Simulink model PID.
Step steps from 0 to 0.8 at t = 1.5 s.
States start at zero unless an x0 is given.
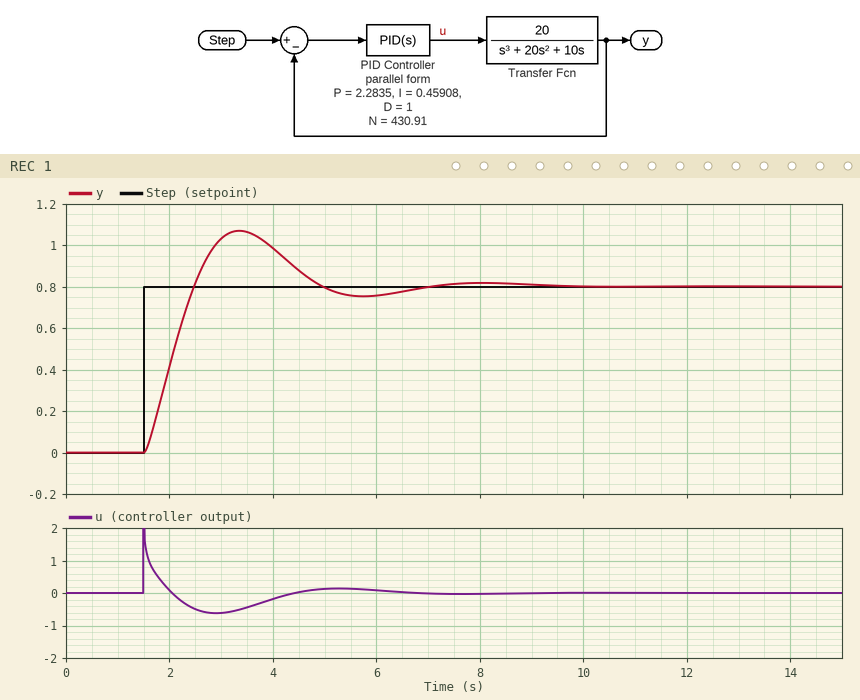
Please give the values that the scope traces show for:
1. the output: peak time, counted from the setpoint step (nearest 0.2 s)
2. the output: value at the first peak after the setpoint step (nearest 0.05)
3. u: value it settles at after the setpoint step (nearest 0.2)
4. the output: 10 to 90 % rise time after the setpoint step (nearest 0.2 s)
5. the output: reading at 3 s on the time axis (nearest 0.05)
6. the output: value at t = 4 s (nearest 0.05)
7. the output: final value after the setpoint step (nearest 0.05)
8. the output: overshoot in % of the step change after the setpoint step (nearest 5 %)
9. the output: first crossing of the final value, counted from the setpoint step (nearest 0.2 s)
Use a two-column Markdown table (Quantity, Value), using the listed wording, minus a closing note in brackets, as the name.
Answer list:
| Quantity | Value |
|---|---|
| the output: peak time, counted from the setpoint step | 1.8 s |
| the output: value at the first peak after the setpoint step | 1.05 |
| u: value it settles at after the setpoint step | 0.0 |
| the output: 10 to 90 % rise time after the setpoint step | 0.8 s |
| the output: reading at 3 s on the time axis | 1.05 |
| the output: value at t = 4 s | 1.00 |
| the output: final value after the setpoint step | 0.80 |
| the output: overshoot in % of the step change after the setpoint step | 35 % |
| the output: first crossing of the final value, counted from the setpoint step | 1.0 s |
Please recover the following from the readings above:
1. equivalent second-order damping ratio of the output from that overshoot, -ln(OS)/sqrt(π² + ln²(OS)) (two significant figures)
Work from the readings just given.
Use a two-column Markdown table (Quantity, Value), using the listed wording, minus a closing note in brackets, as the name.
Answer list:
| Quantity | Value |
|---|---|
| equivalent second-order damping ratio of the output from that overshoot, -ln(OS)/sqrt(π² + ln²(OS)) | 0.32 |
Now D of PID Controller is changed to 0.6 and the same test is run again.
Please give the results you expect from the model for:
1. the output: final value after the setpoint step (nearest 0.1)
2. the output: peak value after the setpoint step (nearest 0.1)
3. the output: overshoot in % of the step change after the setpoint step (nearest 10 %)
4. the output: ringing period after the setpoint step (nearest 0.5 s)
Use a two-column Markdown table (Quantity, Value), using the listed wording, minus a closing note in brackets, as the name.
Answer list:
| Quantity | Value |
|---|---|
| the output: final value after the setpoint step | 0.8 |
| the output: peak value after the setpoint step | 1.2 |
| the output: overshoot in % of the step change after the setpoint step | 50 % |
| the output: ringing period after the setpoint step | 4.5 s |
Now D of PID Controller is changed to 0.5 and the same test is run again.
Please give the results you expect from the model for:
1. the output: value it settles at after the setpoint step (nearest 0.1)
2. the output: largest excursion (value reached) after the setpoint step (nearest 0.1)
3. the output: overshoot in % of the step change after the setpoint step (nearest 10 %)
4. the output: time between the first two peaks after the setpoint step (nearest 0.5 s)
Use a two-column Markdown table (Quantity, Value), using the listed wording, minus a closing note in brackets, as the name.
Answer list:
| Quantity | Value |
|---|---|
| the output: value it settles at after the setpoint step | 0.8 |
| the output: largest excursion (value reached) after the setpoint step | 1.2 |
| the output: overshoot in % of the step change after the setpoint step | 50 % |
| the output: time between the first two peaks after the setpoint step | 4.5 s |
